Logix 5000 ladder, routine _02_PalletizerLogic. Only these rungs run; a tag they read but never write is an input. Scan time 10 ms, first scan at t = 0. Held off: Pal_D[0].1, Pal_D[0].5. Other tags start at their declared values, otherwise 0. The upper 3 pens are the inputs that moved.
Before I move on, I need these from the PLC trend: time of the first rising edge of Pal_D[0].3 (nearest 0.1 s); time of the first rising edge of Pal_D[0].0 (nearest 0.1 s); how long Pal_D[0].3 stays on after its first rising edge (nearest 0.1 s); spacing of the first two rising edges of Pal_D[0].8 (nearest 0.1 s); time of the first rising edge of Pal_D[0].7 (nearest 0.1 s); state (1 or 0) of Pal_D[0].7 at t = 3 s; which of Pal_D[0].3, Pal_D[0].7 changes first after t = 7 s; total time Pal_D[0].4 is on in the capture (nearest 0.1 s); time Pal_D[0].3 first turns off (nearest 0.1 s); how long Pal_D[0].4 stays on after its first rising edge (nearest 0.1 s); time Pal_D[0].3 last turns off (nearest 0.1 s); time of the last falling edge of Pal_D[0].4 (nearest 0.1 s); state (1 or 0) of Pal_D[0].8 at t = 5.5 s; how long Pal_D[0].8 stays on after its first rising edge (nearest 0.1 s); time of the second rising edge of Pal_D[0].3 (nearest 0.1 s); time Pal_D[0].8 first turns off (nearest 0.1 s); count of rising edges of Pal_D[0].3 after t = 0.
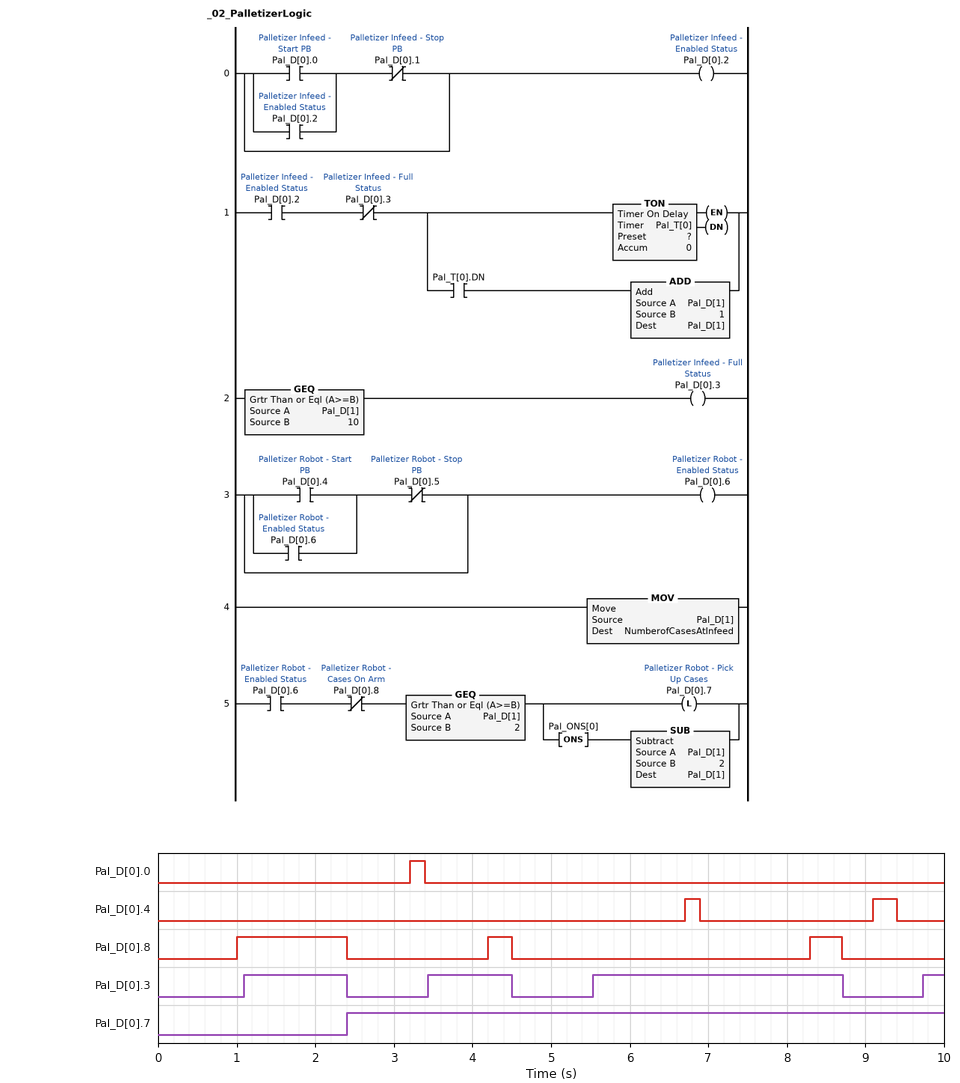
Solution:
1.1 s
3.2 s
1.3 s
3.2 s
2.4 s
1
Pal_D[0].3
0.5 s
2.4 s
0.2 s
8.7 s
9.4 s
0
1.4 s
3.4 s
2.4 s
4
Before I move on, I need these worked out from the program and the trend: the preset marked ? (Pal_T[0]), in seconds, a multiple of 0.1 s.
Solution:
1.0 s
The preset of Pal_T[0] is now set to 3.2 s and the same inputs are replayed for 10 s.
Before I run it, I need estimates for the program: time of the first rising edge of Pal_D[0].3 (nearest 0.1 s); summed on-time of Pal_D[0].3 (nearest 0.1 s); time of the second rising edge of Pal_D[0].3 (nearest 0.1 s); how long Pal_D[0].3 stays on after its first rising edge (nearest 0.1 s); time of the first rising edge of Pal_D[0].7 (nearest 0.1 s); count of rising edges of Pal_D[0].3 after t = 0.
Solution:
4.3 s
1.2 s
7.7 s
0.2 s
3.2 s
2
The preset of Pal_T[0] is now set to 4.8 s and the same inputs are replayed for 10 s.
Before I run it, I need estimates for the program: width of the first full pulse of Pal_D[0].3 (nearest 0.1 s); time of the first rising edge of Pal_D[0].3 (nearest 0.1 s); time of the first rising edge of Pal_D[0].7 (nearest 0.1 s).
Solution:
0.3 s
8.4 s
4.8 s
